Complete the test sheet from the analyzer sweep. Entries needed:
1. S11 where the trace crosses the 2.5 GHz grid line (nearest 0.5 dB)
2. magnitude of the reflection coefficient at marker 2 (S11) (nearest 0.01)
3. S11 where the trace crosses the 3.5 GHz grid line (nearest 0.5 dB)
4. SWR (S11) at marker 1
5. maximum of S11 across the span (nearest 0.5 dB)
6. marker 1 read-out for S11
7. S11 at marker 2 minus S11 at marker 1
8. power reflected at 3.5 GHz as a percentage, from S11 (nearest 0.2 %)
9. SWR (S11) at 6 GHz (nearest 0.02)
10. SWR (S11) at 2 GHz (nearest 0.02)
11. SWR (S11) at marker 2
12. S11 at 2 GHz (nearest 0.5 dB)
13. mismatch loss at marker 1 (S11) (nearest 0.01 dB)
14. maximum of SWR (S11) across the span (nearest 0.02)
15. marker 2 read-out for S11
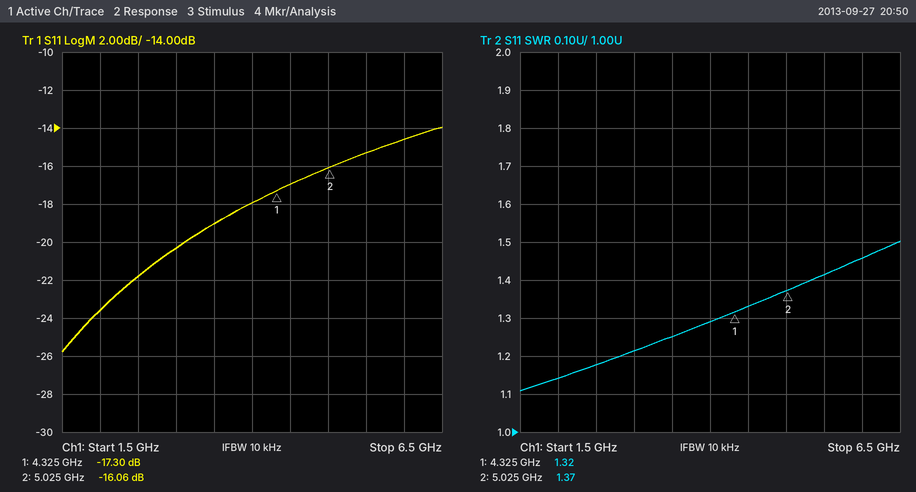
-22.0 dB
0.16
-19.0 dB
1.32
-14.0 dB
-17.30 dB
1.24 dB
1.2 %
1.46
1.14
1.37
-23.5 dB
0.08 dB
1.50
-16.06 dB
